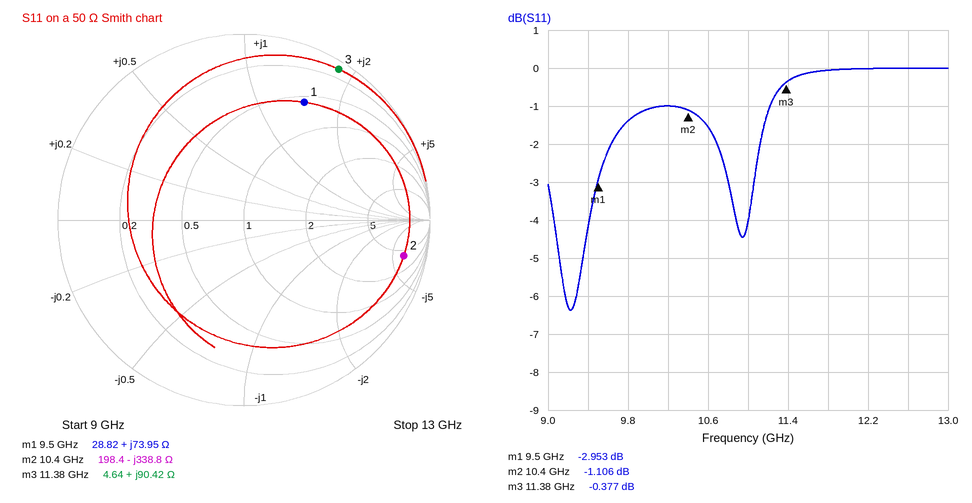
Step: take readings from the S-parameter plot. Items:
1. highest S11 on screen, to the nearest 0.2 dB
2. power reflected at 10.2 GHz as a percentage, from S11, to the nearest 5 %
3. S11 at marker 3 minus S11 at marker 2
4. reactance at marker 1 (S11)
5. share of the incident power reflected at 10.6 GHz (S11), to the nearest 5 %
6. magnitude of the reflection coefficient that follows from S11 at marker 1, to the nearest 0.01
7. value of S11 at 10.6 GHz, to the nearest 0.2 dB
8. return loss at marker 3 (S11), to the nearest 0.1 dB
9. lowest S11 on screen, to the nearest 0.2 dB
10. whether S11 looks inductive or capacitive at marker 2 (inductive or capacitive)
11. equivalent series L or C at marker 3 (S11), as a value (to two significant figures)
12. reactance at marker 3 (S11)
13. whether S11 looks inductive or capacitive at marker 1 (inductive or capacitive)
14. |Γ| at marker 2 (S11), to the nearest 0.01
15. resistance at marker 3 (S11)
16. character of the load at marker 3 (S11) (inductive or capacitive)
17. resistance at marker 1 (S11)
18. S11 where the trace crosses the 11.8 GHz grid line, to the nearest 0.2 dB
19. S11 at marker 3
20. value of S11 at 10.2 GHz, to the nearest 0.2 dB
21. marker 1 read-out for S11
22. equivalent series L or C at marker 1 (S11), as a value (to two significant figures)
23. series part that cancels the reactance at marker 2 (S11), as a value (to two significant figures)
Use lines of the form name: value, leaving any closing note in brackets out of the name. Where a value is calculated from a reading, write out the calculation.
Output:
highest S11 on screen, to the nearest 0.2 dB: 0.0 dB
power reflected at 10.2 GHz as a percentage, from S11, to the nearest 5 %: 10^(-1/10) ≈ 79.4 %, so 80 % to the nearest 5 %
S11 at marker 3 minus S11 at marker 2: -0.377 − (-1.106) = 0.729 dB
reactance at marker 1: +73.95 Ω
share of the incident power reflected at 10.6 GHz (S11), to the nearest 5 %: 10^(-1.6/10) ≈ 69.2 %, so 70 % to the nearest 5 %
magnitude of the reflection coefficient that follows from S11 at marker 1, to the nearest 0.01: 10^(-2.953/20) ≈ 0.71
value of S11 at 10.6 GHz, to the nearest 0.2 dB: -1.6 dB
return loss at marker 3 (S11), to the nearest 0.1 dB: 0.4 dB
lowest S11 on screen, to the nearest 0.2 dB: -6.4 dB
whether S11 looks inductive or capacitive at marker 2: capacitive
equivalent series L or C at marker 3 (S11), as a value: L = 90.42 Ω/(2π × 11.38 GHz) ≈ 1.3 nH
reactance at marker 3: +90.42 Ω
whether S11 looks inductive or capacitive at marker 1: inductive
|Γ| at marker 2 (S11), to the nearest 0.01: 0.88
resistance at marker 3: 4.64 Ω
character of the load at marker 3 (S11): inductive
resistance at marker 1: 28.82 Ω
S11 where the trace crosses the 11.8 GHz grid line, to the nearest 0.2 dB: 0.0 dB
S11 at marker 3: -0.377 dB
value of S11 at 10.2 GHz, to the nearest 0.2 dB: -1.0 dB
marker 1 read-out for S11: -2.953 dB
equivalent series L or C at marker 1 (S11), as a value: L = 73.95 Ω/(2π × 9.5 GHz) ≈ 1.2 nH
series part that cancels the reactance at marker 2 (S11), as a value: L = 338.8 Ω/(2π × 10.4 GHz) ≈ 5.2 nH
